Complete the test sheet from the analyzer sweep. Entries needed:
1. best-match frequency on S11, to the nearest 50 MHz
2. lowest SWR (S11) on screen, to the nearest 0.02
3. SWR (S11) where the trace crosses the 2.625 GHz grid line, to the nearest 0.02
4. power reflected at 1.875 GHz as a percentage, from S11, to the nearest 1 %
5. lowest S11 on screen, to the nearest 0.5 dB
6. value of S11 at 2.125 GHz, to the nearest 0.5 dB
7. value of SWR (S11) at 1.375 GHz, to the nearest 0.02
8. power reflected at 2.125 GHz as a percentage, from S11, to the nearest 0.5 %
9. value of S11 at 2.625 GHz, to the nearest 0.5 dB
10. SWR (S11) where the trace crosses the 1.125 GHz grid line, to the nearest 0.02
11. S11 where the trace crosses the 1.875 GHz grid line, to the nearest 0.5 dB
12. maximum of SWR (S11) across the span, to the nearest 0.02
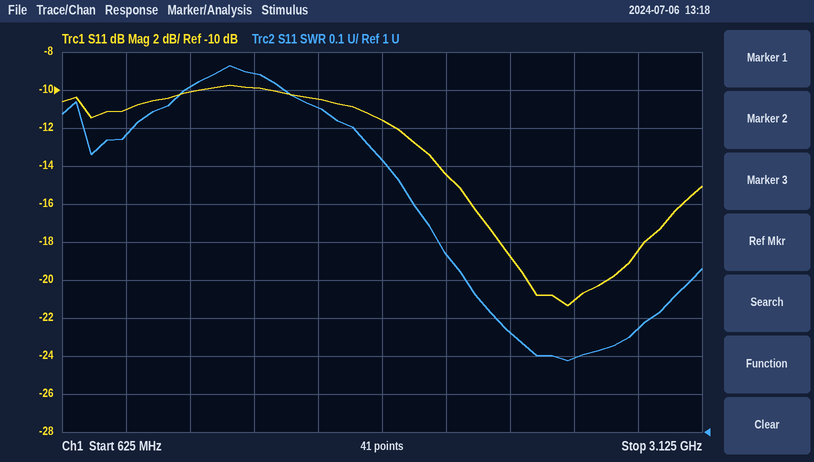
2.60 GHz
1.18
1.20
7 %
-21.5 dB
-14.5 dB
1.94
3.5 %
-21.0 dB
1.90
-11.5 dB
1.96
